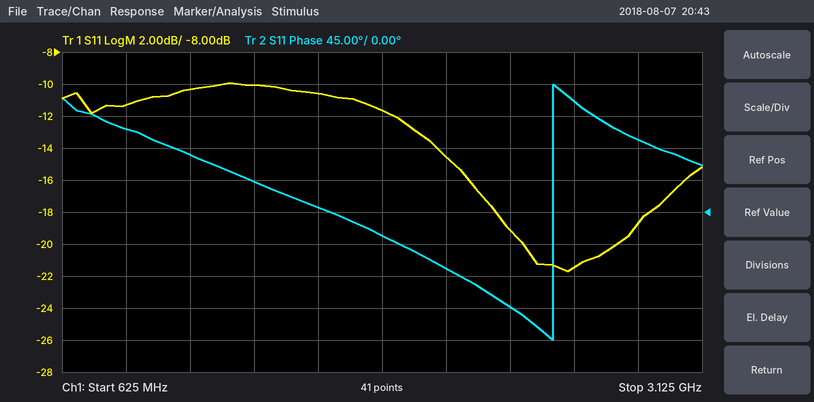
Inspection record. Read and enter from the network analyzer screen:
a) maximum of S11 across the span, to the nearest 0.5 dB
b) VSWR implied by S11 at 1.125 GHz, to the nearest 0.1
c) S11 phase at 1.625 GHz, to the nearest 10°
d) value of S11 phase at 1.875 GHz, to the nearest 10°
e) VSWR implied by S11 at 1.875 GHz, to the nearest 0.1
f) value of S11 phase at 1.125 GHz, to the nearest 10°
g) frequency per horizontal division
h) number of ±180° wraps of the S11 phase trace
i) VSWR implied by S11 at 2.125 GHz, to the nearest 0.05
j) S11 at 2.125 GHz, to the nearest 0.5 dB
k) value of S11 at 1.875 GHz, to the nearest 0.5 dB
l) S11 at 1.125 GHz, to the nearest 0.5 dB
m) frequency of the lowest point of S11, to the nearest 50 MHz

-10.0 dB
1.9
10°
-30°
1.7
80°
250 MHz
1
1.45
-14.5 dB
-11.5 dB
-10.5 dB
2.60 GHz
